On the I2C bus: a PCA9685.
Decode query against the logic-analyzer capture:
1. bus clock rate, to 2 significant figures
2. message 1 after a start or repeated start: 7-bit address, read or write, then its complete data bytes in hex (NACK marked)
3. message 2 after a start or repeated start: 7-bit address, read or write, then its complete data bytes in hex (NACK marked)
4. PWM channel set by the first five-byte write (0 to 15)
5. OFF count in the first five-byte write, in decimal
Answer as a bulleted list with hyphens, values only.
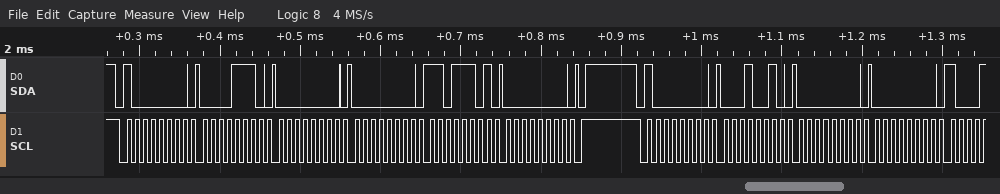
- 100 kHz
- 0x40 write: 0E 00 00 DD 00
- 0x40 write: 12 00 00
- 2
- 221
